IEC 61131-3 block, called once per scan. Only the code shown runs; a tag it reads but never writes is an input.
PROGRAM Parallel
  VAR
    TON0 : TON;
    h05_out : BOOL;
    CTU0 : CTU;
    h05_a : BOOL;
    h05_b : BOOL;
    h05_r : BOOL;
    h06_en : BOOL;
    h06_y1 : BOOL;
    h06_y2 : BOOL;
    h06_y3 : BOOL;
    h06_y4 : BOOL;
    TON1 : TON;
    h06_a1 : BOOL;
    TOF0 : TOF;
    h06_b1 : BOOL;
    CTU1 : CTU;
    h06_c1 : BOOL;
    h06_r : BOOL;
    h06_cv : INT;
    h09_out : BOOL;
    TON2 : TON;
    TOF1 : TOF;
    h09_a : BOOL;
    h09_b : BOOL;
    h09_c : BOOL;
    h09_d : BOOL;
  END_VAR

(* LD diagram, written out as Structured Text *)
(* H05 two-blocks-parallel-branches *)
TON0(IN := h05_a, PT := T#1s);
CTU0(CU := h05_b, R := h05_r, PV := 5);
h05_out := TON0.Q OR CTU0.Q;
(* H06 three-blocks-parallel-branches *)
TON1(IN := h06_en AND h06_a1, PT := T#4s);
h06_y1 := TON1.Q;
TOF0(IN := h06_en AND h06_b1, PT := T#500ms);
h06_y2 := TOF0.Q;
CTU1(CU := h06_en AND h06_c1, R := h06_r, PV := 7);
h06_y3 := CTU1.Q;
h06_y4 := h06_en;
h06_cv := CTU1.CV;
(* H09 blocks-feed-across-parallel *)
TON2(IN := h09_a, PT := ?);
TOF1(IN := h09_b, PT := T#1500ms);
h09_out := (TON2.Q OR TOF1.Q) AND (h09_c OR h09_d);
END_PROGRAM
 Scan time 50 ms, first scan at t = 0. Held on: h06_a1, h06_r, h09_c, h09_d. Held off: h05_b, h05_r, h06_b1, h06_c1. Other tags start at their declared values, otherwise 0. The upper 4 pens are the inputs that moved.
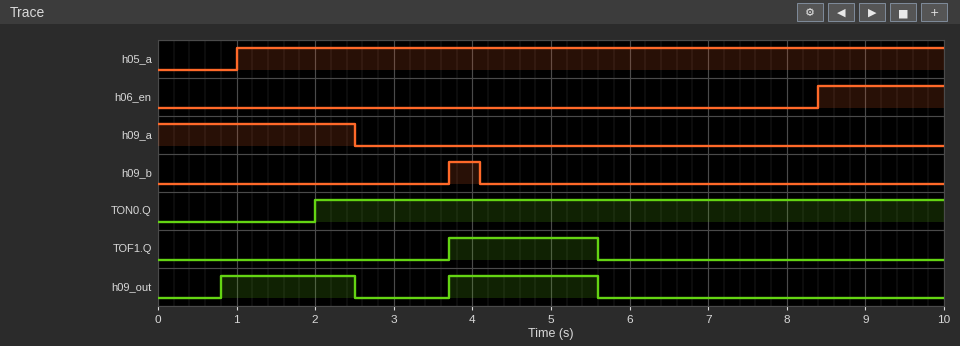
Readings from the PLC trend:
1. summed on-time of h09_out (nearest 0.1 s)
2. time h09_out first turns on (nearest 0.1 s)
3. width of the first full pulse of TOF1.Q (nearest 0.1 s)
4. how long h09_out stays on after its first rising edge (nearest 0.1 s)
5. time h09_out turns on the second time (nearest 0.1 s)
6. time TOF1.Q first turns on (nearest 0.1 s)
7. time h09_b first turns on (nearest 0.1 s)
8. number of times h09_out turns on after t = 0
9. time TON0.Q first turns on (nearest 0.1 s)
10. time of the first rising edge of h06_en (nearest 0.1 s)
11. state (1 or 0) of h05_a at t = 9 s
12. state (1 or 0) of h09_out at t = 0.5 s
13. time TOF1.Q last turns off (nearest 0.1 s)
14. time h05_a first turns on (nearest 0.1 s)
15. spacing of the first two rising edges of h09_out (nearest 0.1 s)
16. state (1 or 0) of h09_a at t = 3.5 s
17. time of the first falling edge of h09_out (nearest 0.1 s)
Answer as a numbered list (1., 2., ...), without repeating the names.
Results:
1. 3.6 s
2. 0.8 s
3. 1.9 s
4. 1.7 s
5. 3.7 s
6. 3.7 s
7. 3.7 s
8. 2
9. 2.0 s
10. 8.4 s
11. 1
12. 0
13. 5.6 s
14. 1.0 s
15. 2.9 s
16. 0
17. 2.5 s
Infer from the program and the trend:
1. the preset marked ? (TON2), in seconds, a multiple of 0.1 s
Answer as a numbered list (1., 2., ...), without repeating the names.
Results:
1. 0.8 s
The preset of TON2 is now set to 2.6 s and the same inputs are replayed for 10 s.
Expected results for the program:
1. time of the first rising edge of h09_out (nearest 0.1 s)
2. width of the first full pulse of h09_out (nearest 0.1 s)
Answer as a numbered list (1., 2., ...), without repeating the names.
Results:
1. 3.7 s
2. 1.9 s
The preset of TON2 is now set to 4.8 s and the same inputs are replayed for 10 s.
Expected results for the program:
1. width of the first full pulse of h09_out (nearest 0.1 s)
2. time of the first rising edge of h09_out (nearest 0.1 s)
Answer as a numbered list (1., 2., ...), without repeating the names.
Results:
1. 1.9 s
2. 3.7 s
